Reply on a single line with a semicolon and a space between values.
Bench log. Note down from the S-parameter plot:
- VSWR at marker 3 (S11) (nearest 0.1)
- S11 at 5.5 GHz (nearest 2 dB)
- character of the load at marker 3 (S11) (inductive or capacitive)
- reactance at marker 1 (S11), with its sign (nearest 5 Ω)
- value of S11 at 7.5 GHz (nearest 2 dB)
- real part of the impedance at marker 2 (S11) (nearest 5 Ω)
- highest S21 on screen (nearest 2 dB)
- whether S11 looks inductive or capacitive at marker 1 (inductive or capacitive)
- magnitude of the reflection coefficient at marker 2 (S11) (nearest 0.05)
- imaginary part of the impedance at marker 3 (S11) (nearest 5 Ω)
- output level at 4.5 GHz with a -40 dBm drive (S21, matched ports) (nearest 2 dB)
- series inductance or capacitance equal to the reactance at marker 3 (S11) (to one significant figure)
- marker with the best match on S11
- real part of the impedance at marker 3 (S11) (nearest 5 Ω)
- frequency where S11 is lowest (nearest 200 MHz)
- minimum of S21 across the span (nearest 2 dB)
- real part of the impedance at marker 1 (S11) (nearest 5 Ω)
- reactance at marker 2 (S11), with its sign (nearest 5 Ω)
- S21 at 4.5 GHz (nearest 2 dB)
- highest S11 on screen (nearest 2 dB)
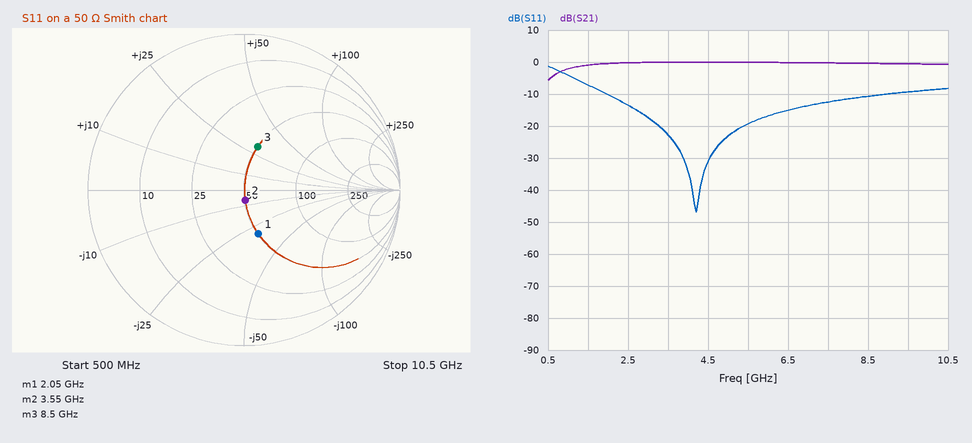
1.8; -20 dB; inductive; -30 Ω; -12 dB; 50 Ω; 0 dB; capacitive; 0.05; +30 Ω; -40 dBm; 600 pH; marker 2; 50 Ω; 4.2 GHz; -6 dB; 50 Ω; -5 Ω; 0 dB; -2 dB
